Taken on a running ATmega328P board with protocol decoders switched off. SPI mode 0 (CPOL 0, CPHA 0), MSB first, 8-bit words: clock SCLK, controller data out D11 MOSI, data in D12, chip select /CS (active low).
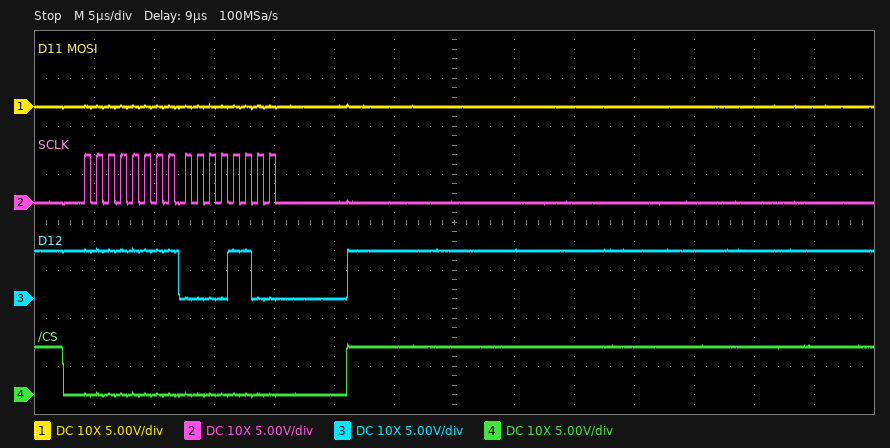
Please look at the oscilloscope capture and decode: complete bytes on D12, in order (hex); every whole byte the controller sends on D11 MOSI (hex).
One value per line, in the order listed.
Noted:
0xFF 0x0C
0x00 0x00
